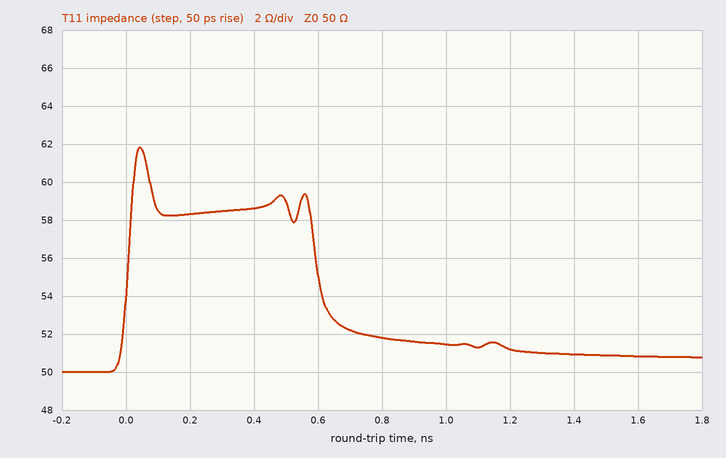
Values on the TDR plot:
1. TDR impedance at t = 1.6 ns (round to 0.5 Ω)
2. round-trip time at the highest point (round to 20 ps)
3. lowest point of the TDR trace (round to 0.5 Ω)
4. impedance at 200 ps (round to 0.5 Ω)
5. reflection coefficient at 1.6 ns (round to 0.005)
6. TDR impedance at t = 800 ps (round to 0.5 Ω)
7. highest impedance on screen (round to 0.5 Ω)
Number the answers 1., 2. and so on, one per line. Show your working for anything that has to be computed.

1. 51.0 Ω
2. 40 ps
3. 50.0 Ω
4. 58.5 Ω
5. (51 − 50)/(51 + 50) ≈ +0.010
6. 52.0 Ω
7. 62.0 Ω
